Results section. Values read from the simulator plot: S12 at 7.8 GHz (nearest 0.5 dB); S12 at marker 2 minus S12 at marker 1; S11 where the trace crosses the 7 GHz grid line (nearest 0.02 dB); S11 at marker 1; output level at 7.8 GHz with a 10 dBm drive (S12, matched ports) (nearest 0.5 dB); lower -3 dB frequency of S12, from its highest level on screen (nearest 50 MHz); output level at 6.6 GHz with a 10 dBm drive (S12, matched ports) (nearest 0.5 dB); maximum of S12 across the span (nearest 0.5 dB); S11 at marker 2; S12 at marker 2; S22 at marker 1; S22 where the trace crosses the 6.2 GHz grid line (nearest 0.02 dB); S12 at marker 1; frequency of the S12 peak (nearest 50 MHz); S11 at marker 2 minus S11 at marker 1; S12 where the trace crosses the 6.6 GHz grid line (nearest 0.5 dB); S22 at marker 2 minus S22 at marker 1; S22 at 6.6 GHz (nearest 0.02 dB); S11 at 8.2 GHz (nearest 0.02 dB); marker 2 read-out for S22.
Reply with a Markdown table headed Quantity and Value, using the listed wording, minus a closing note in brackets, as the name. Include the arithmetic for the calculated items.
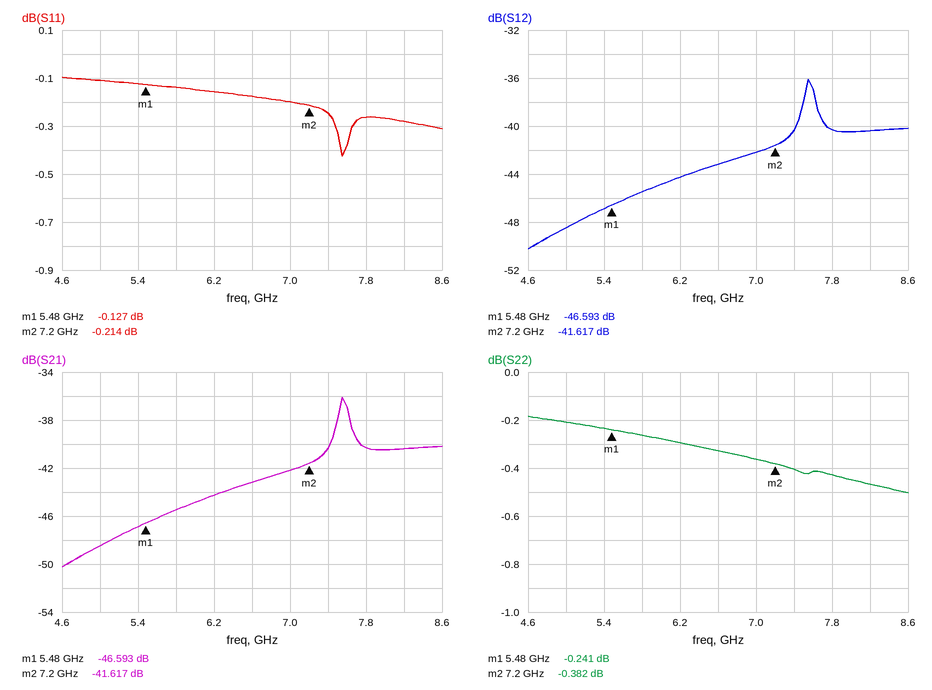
| Quantity | Value |
|---|---|
| S12 at 7.8 GHz | -40.5 dB |
| S12 at marker 2 minus S12 at marker 1 | -41.617 − (-46.593) = 4.976 dB |
| S11 where the trace crosses the 7 GHz grid line | -0.20 dB |
| S11 at marker 1 | -0.127 dB |
| output level at 7.8 GHz with a 10 dBm drive (S12, matched ports) | 10 dBm + (-40.5 dB) = -30.5 dBm |
| lower -3 dB frequency of S12, from its highest level on screen | 7.45 GHz |
| output level at 6.6 GHz with a 10 dBm drive (S12, matched ports) | 10 dBm + (-43.0 dB) = -33.0 dBm |
| maximum of S12 across the span | -36.0 dB |
| S11 at marker 2 | -0.214 dB |
| S12 at marker 2 | -41.617 dB |
| S22 at marker 1 | -0.241 dB |
| S22 where the trace crosses the 6.2 GHz grid line | -0.30 dB |
| S12 at marker 1 | -46.593 dB |
| frequency of the S12 peak | 7.55 GHz |
| S11 at marker 2 minus S11 at marker 1 | -0.214 − (-0.127) = -0.087 dB |
| S12 where the trace crosses the 6.6 GHz grid line | -43.0 dB |
| S22 at marker 2 minus S22 at marker 1 | -0.382 − (-0.241) = -0.141 dB |
| S22 at 6.6 GHz | -0.32 dB |
| S11 at 8.2 GHz | -0.28 dB |
| marker 2 read-out for S22 | -0.382 dB |
